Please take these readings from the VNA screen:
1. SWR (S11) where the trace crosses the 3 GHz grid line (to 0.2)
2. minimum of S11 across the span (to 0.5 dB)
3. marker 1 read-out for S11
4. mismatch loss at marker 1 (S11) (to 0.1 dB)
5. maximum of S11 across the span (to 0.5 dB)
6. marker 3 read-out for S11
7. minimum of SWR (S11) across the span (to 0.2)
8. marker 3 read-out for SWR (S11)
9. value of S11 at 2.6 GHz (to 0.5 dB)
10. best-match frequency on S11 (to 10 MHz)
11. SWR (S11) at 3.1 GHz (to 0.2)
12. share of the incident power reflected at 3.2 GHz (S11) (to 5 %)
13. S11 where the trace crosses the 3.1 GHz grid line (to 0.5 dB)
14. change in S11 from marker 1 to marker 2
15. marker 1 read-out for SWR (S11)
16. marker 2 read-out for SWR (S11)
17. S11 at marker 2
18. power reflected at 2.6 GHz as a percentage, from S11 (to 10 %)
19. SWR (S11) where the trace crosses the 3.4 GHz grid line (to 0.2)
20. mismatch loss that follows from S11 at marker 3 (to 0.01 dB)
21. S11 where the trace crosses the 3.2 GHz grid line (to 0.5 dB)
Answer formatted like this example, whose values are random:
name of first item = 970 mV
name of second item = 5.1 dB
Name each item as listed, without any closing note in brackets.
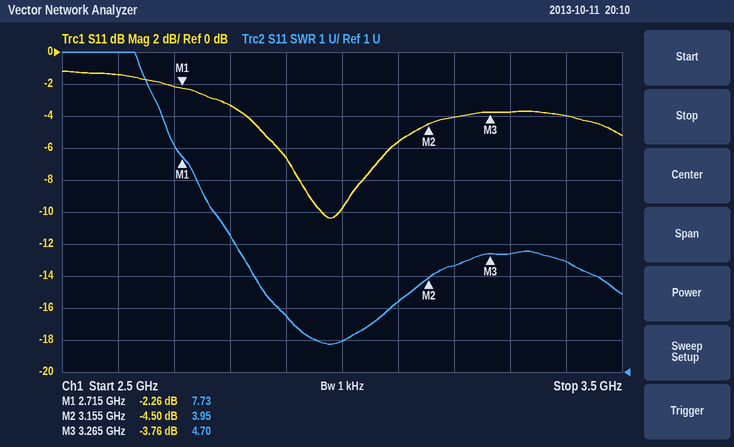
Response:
SWR (S11) where the trace crosses the 3 GHz grid line = 2.0
minimum of S11 across the span = -10.5 dB
marker 1 read-out for S11 = -2.26 dB
mismatch loss at marker 1 (S11) = 3.9 dB
maximum of S11 across the span = -1.0 dB
marker 3 read-out for S11 = -3.76 dB
minimum of SWR (S11) across the span = 1.8
marker 3 read-out for SWR = 4.70
value of S11 at 2.6 GHz = -1.5 dB
best-match frequency on S11 = 2.98 GHz
SWR (S11) at 3.1 GHz = 3.2
share of the incident power reflected at 3.2 GHz (S11) = 40 %
S11 where the trace crosses the 3.1 GHz grid line = -5.5 dB
change in S11 from marker 1 to marker 2 = -2.24 dB
marker 1 read-out for SWR = 7.73
marker 2 read-out for SWR = 3.95
S11 at marker 2 = -4.50 dB
power reflected at 2.6 GHz as a percentage, from S11 = 70 %
SWR (S11) where the trace crosses the 3.4 GHz grid line = 4.4
mismatch loss that follows from S11 at marker 3 = 2.37 dB
S11 where the trace crosses the 3.2 GHz grid line = -4.0 dB
